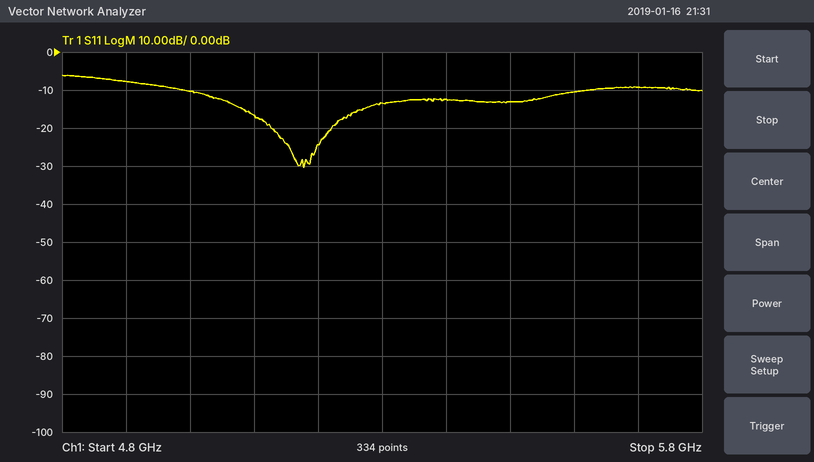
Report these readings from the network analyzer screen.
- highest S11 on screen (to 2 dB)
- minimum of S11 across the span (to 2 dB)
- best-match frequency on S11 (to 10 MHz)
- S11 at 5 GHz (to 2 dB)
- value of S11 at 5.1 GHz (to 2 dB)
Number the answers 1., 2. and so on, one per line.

1. -6 dB
2. -30 dB
3. 5.18 GHz
4. -10 dB
5. -16 dB
